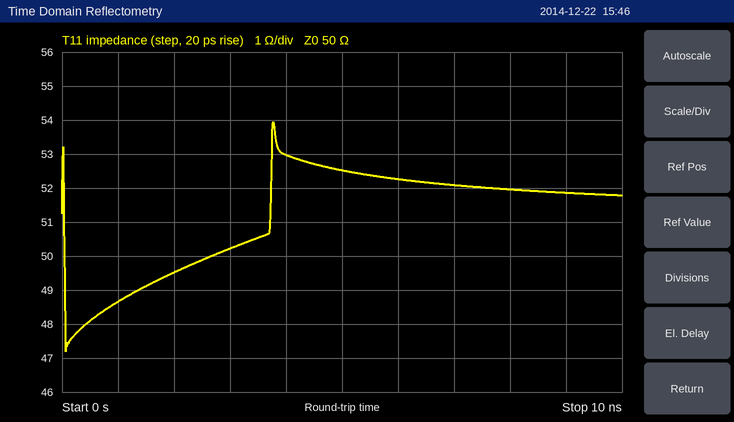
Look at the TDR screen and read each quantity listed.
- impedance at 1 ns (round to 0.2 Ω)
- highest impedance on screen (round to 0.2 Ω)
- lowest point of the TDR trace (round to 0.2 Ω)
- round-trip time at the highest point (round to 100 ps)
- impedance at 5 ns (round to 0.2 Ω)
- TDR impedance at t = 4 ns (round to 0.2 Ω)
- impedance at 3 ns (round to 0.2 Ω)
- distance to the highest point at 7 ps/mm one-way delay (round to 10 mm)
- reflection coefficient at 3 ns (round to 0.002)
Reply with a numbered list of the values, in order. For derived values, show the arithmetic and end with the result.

1. 48.6 Ω
2. 54.0 Ω
3. 47.2 Ω
4. 3.8 ns
5. 52.6 Ω
6. 53.0 Ω
7. 50.2 Ω
8. 3.8 ns / 2 / 7 ps/mm ≈ 271 mm, so 270 mm to the nearest 10 mm
9. (50.2 − 50)/(50.2 + 50) ≈ +0.002
